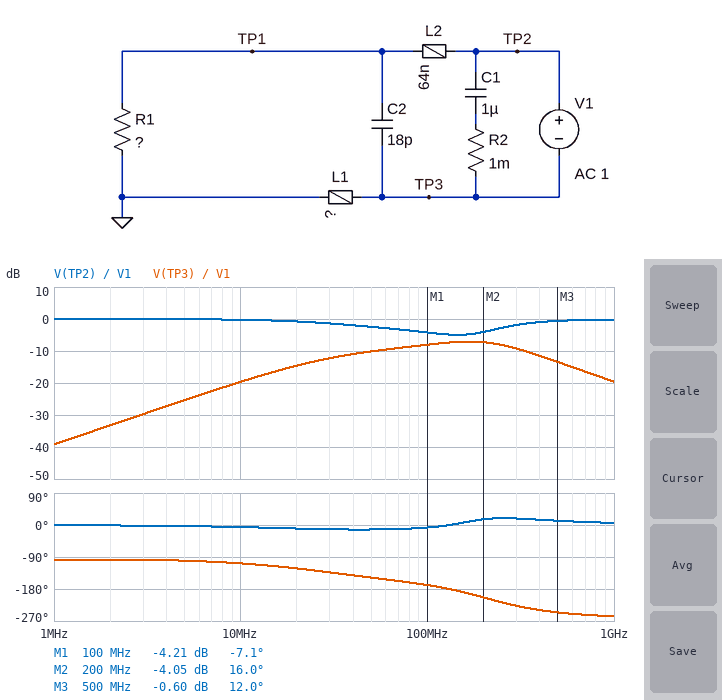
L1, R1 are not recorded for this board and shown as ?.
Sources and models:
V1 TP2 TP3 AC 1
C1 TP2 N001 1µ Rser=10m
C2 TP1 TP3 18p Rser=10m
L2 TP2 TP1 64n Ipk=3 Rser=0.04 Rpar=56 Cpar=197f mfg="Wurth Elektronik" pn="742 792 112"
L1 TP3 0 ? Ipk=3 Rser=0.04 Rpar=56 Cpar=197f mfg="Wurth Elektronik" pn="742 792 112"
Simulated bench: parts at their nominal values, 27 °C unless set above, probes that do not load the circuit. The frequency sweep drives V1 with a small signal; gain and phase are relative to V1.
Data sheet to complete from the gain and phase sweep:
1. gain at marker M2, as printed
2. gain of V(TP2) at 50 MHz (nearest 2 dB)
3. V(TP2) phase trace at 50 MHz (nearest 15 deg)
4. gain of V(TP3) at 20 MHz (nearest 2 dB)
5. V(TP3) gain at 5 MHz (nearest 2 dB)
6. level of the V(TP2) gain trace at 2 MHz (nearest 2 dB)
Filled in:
-4.05 dB
-2 dB
-15 deg
-14 dB
-26 dB
0 dB
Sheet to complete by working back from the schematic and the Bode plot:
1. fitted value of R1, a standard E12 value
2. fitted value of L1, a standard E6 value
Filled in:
27 Ω
47 nH
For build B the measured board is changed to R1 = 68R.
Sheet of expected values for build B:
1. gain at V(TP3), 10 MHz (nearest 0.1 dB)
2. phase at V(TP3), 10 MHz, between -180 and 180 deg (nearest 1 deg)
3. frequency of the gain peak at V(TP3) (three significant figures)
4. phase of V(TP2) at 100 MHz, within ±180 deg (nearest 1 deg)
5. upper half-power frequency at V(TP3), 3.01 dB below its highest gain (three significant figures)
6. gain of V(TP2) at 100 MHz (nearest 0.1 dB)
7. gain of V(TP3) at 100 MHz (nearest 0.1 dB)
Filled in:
-27.3 dB
-100 deg
158 MHz
-8 deg
310 MHz
-2.6 dB
-11.0 dB
